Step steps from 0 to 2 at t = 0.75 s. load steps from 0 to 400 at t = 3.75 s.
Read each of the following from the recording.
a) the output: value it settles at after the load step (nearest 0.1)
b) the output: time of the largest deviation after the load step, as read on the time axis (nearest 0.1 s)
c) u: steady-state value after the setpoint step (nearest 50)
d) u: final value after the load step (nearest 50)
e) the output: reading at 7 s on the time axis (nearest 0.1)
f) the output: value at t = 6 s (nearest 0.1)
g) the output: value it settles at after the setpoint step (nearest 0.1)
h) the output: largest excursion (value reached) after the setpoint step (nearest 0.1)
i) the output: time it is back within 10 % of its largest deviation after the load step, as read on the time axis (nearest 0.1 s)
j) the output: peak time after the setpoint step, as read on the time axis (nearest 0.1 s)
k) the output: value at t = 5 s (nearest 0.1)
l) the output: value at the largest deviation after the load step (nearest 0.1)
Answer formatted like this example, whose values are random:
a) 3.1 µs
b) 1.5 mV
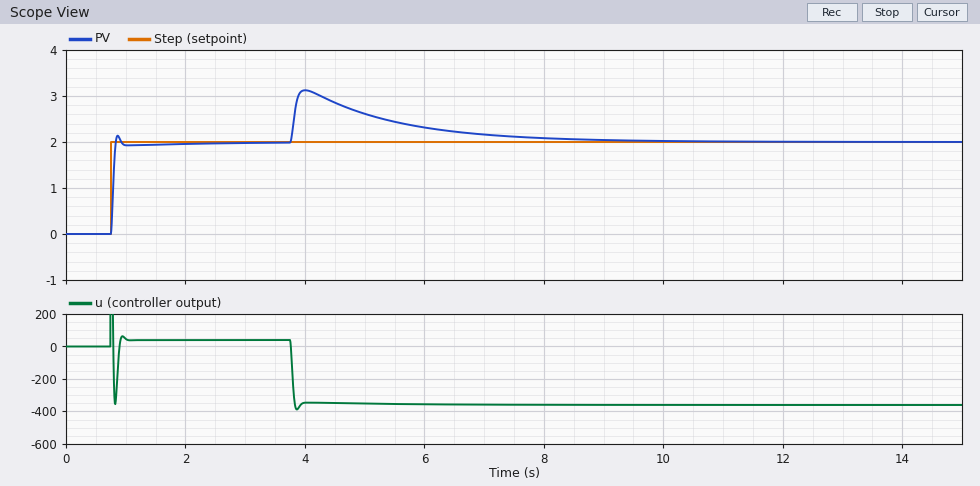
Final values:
a) 2.0
b) 4.0 s
c) 50
d) -350
e) 2.2
f) 2.3
g) 2.0
h) 2.1
i) 7.5 s
j) 0.9 s
k) 2.6
l) 3.1
